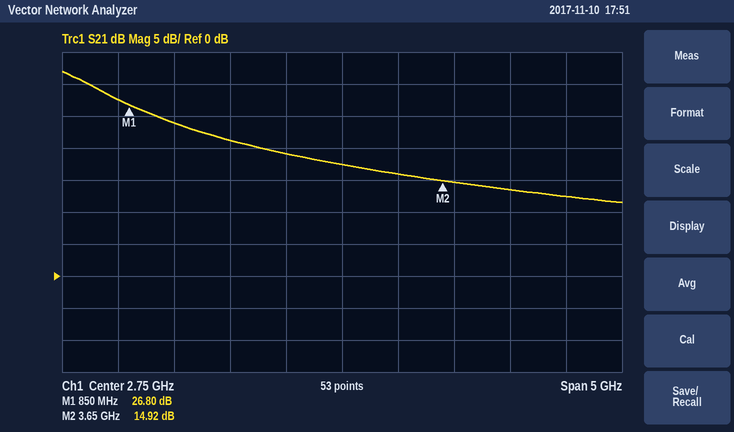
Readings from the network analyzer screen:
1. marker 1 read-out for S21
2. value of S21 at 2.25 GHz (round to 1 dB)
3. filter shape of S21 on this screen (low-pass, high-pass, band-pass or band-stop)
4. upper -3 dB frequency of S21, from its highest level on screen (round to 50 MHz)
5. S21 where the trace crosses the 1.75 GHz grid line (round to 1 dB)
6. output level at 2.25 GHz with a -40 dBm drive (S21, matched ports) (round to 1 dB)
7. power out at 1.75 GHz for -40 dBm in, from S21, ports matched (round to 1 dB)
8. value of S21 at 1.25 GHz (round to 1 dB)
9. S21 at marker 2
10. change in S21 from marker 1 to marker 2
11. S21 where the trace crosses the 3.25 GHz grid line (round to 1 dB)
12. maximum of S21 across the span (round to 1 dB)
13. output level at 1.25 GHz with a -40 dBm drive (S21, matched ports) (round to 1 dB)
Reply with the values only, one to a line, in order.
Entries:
26.80 dB
19 dB
low-pass
600 MHz
21 dB
-21 dBm
-19 dBm
24 dB
14.92 dB
-11.88 dB
16 dB
32 dB
-16 dBm
